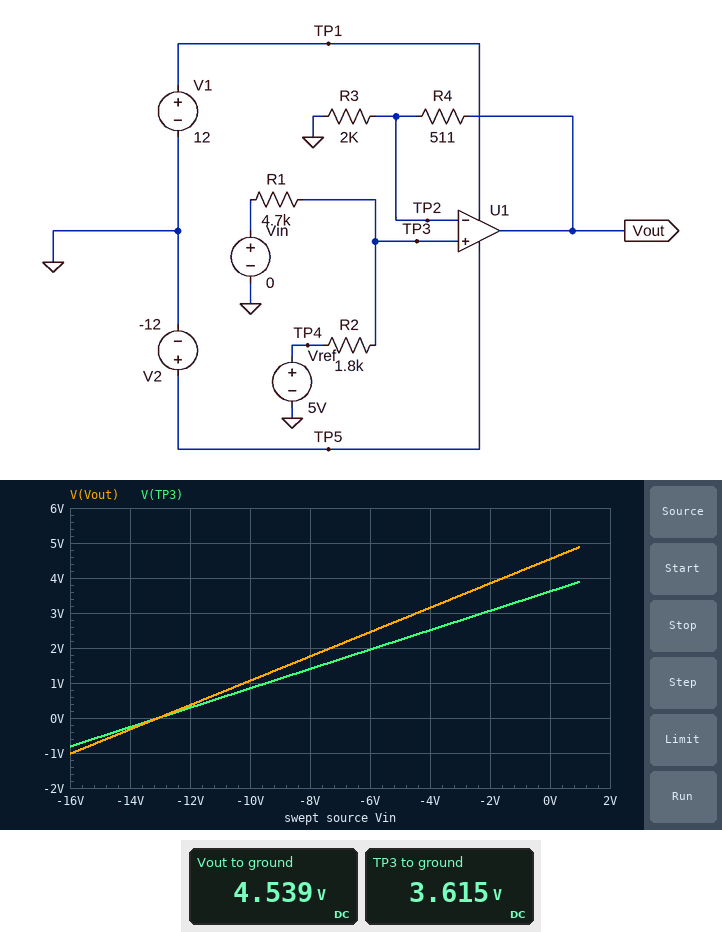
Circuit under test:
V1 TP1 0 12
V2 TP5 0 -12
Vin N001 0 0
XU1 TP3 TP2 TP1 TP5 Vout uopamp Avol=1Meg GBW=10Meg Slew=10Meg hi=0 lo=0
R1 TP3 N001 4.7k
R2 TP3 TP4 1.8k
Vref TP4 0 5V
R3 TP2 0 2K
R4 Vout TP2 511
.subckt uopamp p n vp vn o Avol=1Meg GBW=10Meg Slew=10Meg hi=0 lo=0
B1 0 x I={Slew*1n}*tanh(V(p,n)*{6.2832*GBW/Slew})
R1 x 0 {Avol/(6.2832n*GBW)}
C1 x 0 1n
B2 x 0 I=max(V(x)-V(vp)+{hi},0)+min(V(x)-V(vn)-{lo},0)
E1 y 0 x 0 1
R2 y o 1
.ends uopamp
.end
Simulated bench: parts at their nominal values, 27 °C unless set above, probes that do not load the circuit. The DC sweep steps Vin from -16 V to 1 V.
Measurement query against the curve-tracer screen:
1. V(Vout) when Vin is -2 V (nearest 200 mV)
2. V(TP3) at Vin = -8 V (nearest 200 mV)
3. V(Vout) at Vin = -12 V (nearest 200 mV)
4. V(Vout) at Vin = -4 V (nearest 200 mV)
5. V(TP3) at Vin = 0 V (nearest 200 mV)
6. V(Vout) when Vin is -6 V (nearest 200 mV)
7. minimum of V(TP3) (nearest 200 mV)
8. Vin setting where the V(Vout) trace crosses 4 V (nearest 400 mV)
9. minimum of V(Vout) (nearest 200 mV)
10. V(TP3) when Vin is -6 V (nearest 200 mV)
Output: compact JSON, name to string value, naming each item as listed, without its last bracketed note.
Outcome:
{"V(Vout) when Vin is -2 V": "3.8 V", "V(TP3) at Vin = -8 V": "1.4 V", "V(Vout) at Vin = -12 V": "400 mV", "V(Vout) at Vin = -4 V": "3.2 V", "V(TP3) at Vin = 0 V": "3.6 V", "V(Vout) when Vin is -6 V": "2.4 V", "minimum of V(TP3)": "-800 mV", "Vin setting where the V(Vout) trace crosses 4 V": "-1.6 V", "minimum of V(Vout)": "-1.0 V", "V(TP3) when Vin is -6 V": "2.0 V"}
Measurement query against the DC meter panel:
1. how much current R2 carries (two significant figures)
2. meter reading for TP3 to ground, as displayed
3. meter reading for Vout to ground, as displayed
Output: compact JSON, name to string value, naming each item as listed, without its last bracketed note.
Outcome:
{"how much current R2 carries": "770 µA", "meter reading for TP3 to ground, as displayed": "3.615 V", "meter reading for Vout to ground, as displayed": "4.539 V"}
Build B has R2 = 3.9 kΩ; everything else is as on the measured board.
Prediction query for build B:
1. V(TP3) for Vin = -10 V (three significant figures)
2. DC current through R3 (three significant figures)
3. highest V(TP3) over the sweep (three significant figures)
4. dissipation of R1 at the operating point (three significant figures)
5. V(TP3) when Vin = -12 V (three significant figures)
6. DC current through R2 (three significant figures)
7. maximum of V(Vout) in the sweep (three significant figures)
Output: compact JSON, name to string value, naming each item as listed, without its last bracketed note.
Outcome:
{"V(TP3) for Vin = -10 V": "-1.80 V", "DC current through R3": "1.37 mA", "highest V(TP3) over the sweep": "3.19 V", "dissipation of R1 at the operating point": "1.59 mW", "V(TP3) when Vin = -12 V": "-2.71 V", "DC current through R2": "581 µA", "maximum of V(Vout) in the sweep": "4.00 V"}
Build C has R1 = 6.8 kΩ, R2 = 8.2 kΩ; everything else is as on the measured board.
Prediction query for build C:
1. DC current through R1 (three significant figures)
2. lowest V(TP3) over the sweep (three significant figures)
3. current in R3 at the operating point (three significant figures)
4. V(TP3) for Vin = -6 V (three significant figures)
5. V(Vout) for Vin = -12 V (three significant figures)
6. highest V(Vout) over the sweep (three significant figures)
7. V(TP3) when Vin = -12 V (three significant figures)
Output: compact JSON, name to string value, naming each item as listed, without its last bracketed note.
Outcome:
{"DC current through R1": "333 µA", "lowest V(TP3) over the sweep": "-6.48 V", "current in R3 at the operating point": "1.13 mA", "V(TP3) for Vin = -6 V": "-1.01 V", "V(Vout) for Vin = -12 V": "-5.39 V", "highest V(Vout) over the sweep": "3.53 V", "V(TP3) when Vin = -12 V": "-4.29 V"}
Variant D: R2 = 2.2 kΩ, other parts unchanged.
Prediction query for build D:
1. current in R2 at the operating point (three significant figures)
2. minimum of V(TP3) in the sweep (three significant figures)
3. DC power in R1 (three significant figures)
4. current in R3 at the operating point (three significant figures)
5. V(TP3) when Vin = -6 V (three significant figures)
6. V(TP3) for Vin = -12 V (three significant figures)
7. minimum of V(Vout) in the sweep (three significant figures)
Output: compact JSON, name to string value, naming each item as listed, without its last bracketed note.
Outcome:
{"current in R2 at the operating point": "725 µA", "minimum of V(TP3) in the sweep": "-1.70 V", "DC power in R1": "2.47 mW", "current in R3 at the operating point": "1.70 mA", "V(TP3) when Vin = -6 V": "1.49 V", "V(TP3) for Vin = -12 V": "-420 mV", "minimum of V(Vout) in the sweep": "-2.13 V"}
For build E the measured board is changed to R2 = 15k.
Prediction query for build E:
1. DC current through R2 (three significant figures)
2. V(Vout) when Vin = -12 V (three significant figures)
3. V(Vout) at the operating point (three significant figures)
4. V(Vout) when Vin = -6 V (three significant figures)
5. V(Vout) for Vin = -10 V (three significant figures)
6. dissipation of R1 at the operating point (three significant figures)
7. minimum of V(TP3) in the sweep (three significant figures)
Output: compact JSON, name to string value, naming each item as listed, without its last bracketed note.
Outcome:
{"DC current through R2": "254 µA", "V(Vout) when Vin = -12 V": "-9.97 V", "V(Vout) at the operating point": "1.50 V", "V(Vout) when Vin = -6 V": "-4.24 V", "V(Vout) for Vin = -10 V": "-8.06 V", "dissipation of R1 at the operating point": "303 µW", "minimum of V(TP3) in the sweep": "-11.0 V"}
